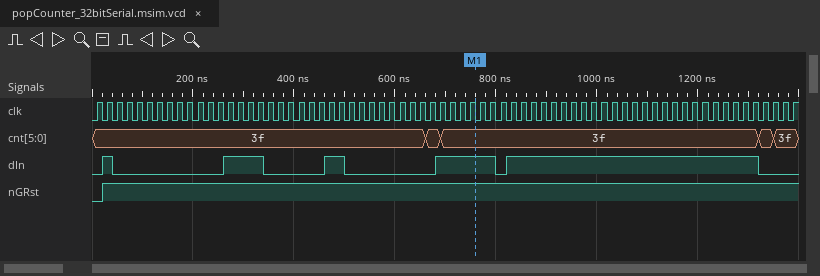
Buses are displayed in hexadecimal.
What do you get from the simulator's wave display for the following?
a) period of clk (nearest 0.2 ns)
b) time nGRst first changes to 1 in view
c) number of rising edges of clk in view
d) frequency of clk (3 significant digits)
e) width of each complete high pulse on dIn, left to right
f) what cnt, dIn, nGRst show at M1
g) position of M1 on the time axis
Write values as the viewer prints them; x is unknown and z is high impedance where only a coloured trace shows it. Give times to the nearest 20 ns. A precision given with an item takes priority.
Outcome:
20 ns
20 ns
70
50.0 MHz
20 ns, 80 ns, 40 ns, 120 ns, 500 ns
cnt=3f, dIn=1, nGRst=1
760 ns
